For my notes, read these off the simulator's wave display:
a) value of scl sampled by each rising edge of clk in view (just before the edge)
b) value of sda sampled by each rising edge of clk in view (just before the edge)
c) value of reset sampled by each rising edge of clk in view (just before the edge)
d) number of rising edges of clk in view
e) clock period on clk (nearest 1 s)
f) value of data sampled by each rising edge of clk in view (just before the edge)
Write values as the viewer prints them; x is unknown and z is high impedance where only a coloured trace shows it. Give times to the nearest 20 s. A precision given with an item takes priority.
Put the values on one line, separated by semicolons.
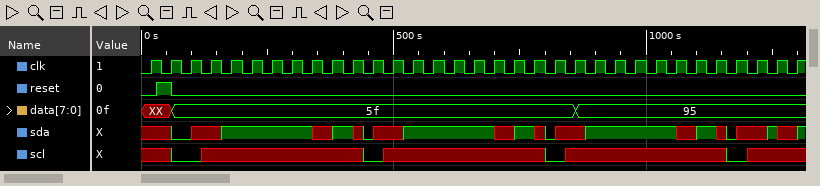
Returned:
x x 0 x x x x x x x x 0 x x x x x x x x 0 x x x x x x x x 0 x x x; x x 0 x 1 1 1 1 1 x 1 0 x 1 1 1 1 1 x 1 0 x 1 1 1 1 1 x 1 0 x 1 x; 0 1 0 0 0 0 0 0 0 0 0 0 0 0 0 0 0 0 0 0 0 0 0 0 0 0 0 0 0 0 0 0 0; 33; 40 s; XX, XX, 5f, 5f, 5f, 5f, 5f, 5f, 5f, 5f, 5f, 5f, 5f, 5f, 5f, 5f, 5f, 5f, 5f, 5f, 5f, 5f, 95, 95, 95, 95, 95, 95, 95, 95, 95, 95, 95
